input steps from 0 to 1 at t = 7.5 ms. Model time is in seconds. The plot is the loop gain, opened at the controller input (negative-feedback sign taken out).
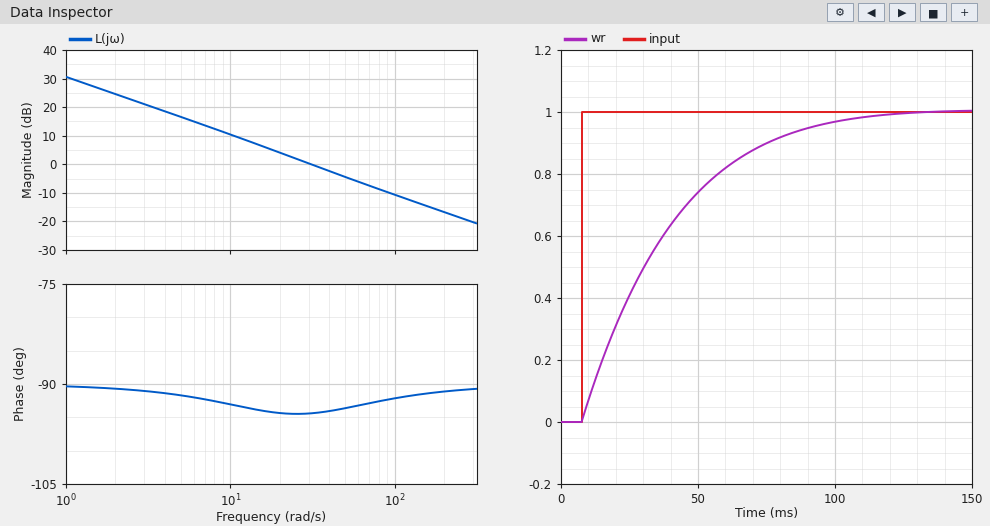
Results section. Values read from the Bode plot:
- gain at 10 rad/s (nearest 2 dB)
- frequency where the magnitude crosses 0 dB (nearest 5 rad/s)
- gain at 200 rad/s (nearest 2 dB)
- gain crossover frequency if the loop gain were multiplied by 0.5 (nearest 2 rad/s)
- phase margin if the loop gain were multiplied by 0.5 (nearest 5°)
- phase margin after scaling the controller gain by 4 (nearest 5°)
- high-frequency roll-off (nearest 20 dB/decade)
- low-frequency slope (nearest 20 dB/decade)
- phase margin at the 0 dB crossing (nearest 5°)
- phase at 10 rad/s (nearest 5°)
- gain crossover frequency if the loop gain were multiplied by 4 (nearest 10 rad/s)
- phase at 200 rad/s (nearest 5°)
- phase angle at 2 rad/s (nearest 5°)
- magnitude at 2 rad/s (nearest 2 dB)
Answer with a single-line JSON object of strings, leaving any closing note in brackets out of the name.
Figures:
{"gain at 10 rad/s": "10 dB", "frequency where the magnitude crosses 0 dB": "30 rad/s", "gain at 200 rad/s": "-16 dB", "gain crossover frequency if the loop gain were multiplied by 0.5": "16 rad/s", "phase margin if the loop gain were multiplied by 0.5": "85°", "phase margin after scaling the controller gain by 4": "90°", "high-frequency roll-off": "-20 dB/decade", "low-frequency slope": "-20 dB/decade", "phase margin at the 0 dB crossing": "85°", "phase at 10 rad/s": "-95°", "gain crossover frequency if the loop gain were multiplied by 4": "120 rad/s", "phase at 200 rad/s": "-90°", "phase angle at 2 rad/s": "-90°", "magnitude at 2 rad/s": "24 dB"}
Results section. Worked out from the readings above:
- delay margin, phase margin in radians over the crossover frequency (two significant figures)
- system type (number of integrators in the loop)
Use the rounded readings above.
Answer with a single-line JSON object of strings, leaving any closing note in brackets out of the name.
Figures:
{"delay margin, phase margin in radians over the crossover frequency": "0.049 s", "system type": "1"}
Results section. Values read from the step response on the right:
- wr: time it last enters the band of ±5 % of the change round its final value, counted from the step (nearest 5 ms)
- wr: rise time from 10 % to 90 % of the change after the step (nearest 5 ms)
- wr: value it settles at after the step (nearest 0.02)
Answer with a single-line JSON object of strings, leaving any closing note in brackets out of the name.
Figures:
{"wr: time it last enters the band of ±5 % of the change round its final value, counted from the step": "85 ms", "wr: rise time from 10 % to 90 % of the change after the step": "65 ms", "wr: value it settles at after the step": "1.00"}
